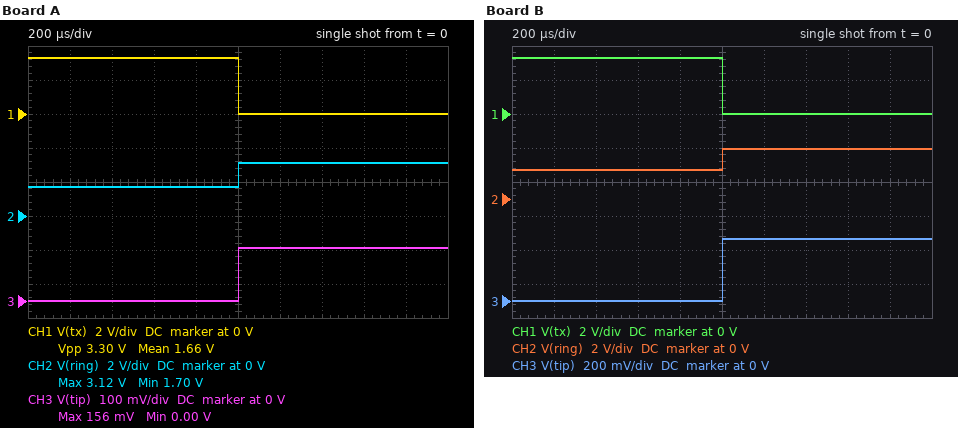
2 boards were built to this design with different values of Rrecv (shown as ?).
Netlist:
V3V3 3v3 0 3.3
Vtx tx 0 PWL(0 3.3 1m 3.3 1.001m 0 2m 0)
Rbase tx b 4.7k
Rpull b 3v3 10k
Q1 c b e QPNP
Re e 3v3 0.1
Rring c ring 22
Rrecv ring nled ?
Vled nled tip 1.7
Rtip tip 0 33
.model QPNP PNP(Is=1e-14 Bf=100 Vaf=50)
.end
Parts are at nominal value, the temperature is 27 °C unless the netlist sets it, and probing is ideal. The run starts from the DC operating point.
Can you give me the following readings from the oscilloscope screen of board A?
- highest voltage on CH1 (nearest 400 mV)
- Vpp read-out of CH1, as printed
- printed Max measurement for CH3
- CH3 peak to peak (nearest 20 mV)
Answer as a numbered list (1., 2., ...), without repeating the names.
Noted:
1. 3.2 V
2. 3.30 V
3. 156 mV
4. 160 mV
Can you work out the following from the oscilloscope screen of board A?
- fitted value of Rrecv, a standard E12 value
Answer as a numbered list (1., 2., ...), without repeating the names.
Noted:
1. 270 Ω
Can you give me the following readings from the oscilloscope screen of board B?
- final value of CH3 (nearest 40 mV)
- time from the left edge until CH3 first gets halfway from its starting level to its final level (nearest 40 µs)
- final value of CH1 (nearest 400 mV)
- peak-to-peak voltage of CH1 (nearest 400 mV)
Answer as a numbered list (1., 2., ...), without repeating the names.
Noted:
1. 360 mV
2. 1.00 ms
3. 0 V
4. 3.2 V
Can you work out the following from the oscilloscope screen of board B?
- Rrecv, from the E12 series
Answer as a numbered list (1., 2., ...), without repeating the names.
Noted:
1. 82 Ω
